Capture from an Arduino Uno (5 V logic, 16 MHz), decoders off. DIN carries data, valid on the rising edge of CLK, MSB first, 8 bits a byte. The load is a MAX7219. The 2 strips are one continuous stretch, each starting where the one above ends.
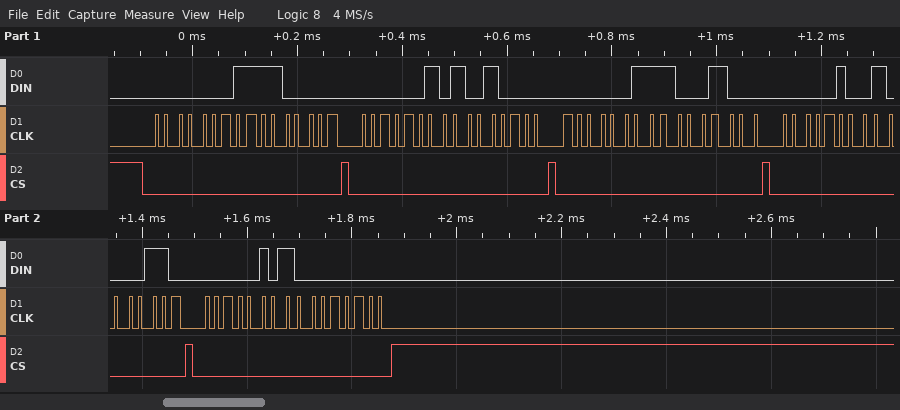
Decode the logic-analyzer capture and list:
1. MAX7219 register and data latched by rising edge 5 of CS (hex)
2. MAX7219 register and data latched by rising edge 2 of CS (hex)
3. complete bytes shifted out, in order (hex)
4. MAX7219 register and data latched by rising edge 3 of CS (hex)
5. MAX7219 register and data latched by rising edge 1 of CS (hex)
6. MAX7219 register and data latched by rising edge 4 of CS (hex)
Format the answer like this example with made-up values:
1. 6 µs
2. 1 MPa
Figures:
1. register 0x5, data 0x00
2. register 0x2, data 0x90
3. 01 E0 02 90 03 88 04 86 05 00
4. register 0x3, data 0x88
5. register 0x1, data 0xE0
6. register 0x4, data 0x86
